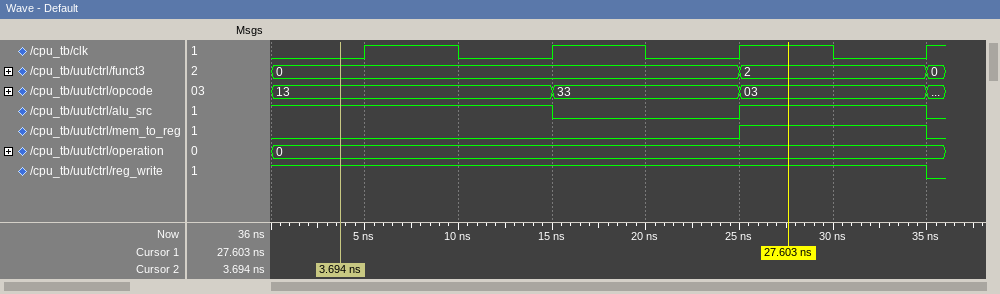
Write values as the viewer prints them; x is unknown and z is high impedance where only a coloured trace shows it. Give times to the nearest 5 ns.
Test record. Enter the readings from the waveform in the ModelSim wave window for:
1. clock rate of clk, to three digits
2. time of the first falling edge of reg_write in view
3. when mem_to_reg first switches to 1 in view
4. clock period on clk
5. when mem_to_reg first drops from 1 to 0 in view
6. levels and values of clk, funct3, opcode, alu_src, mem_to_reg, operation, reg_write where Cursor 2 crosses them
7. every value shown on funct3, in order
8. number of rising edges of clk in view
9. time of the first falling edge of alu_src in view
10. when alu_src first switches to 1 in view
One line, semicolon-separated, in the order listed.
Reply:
100 MHz; 35 ns; 25 ns; 10 ns; 35 ns; clk=0, funct3=0, opcode=13, alu_src=1, mem_to_reg=0, operation=0, reg_write=1; 0, 2, 0; 4; 15 ns; 25 ns
